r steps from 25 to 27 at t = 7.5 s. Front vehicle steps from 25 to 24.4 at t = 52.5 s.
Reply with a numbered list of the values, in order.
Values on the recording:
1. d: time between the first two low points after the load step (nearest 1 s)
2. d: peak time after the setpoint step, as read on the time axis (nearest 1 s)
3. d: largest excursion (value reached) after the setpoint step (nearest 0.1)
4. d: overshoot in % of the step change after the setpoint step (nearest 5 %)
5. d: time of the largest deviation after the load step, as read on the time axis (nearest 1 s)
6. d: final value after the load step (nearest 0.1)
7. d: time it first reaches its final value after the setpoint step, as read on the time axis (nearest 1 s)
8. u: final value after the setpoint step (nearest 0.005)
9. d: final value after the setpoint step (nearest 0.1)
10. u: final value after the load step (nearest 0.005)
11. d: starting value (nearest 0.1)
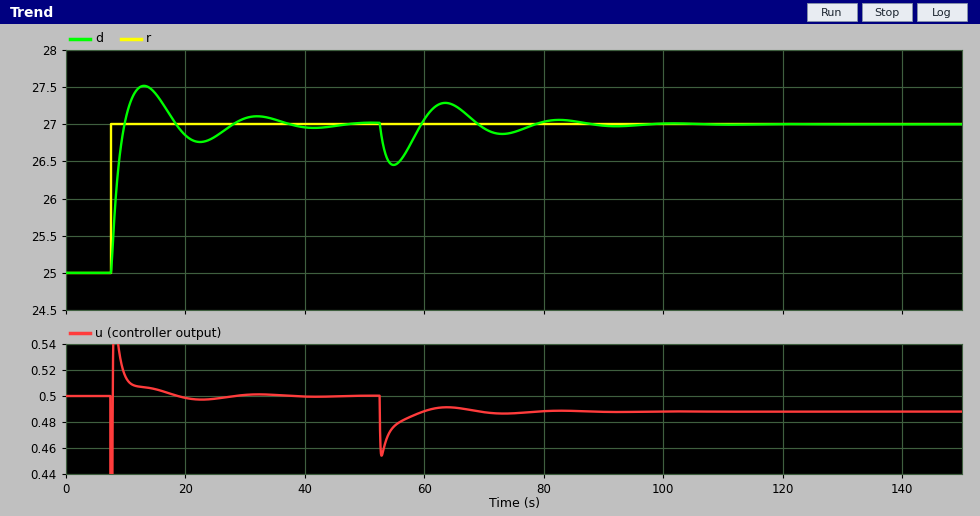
1. 18 s
2. 13 s
3. 27.5
4. 25 %
5. 55 s
6. 27.0
7. 10 s
8. 0.500
9. 27.0
10. 0.490
11. 25.0
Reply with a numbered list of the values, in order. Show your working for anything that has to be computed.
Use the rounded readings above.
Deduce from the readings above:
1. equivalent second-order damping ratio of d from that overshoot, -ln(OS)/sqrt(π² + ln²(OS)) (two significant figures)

1. ln(0.25) = -1.386; 1.386 / sqrt(9.870 + 1.922) = 0.40
